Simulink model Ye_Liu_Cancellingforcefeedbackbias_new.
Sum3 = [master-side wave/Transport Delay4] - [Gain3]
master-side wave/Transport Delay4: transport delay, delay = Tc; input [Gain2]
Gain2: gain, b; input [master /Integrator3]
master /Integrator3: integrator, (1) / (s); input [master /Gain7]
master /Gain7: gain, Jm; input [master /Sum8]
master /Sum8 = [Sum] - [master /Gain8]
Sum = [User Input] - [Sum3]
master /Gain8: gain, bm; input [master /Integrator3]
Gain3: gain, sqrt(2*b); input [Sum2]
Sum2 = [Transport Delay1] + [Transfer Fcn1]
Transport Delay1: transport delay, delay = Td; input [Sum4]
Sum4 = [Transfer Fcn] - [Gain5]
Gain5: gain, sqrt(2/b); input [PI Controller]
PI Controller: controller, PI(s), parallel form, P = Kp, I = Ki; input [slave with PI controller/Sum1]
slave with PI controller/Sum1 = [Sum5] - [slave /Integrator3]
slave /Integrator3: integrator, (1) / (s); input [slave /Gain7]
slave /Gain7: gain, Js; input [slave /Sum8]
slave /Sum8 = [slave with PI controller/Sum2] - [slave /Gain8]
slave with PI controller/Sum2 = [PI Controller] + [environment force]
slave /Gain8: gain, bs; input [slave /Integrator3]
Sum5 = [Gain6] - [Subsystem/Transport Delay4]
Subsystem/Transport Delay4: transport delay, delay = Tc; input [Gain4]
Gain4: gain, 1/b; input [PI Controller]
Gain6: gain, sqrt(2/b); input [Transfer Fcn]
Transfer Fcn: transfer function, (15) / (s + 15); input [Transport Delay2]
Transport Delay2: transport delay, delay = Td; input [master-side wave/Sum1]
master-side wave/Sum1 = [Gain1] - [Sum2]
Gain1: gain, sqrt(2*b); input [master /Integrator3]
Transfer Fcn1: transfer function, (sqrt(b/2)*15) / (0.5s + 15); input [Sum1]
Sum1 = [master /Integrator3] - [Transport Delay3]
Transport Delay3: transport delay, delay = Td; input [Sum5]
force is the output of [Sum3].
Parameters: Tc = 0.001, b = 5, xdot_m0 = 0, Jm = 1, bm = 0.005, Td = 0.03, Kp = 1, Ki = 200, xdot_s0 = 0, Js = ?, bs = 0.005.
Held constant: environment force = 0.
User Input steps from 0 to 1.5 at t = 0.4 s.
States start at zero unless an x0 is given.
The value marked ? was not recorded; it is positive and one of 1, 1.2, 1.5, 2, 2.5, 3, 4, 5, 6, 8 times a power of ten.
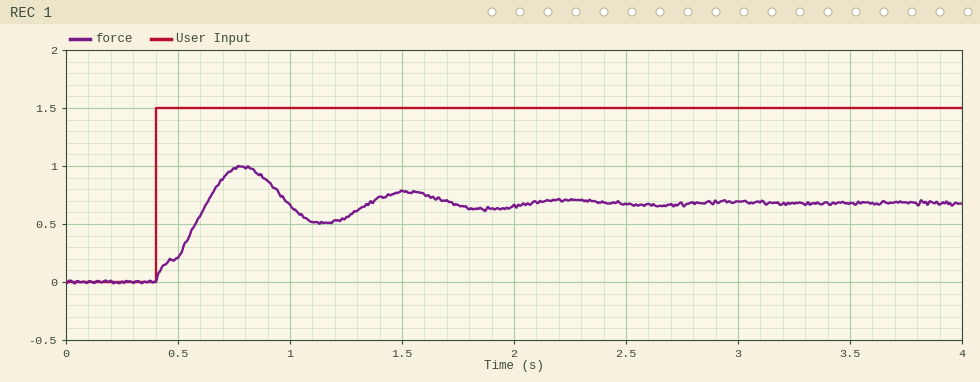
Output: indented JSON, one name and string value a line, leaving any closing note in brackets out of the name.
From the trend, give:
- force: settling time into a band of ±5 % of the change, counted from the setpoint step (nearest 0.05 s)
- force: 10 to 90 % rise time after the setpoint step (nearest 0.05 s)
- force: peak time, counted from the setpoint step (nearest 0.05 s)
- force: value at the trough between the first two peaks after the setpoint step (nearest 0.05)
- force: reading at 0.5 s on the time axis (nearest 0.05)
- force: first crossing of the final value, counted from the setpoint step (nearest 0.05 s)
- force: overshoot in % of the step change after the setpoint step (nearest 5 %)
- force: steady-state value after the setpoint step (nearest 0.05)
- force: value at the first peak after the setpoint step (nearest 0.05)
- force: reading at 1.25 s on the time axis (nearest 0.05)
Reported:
{
  "force: settling time into a band of ±5 % of the change, counted from the setpoint step": "1.60 s",
  "force: 10 to 90 % rise time after the setpoint step": "0.20 s",
  "force: peak time, counted from the setpoint step": "0.40 s",
  "force: value at the trough between the first two peaks after the setpoint step": "0.50",
  "force: reading at 0.5 s on the time axis": "0.20",
  "force: first crossing of the final value, counted from the setpoint step": "0.25 s",
  "force: overshoot in % of the step change after the setpoint step": "45 %",
  "force: steady-state value after the setpoint step": "0.70",
  "force: value at the first peak after the setpoint step": "1.00",
  "force: reading at 1.25 s on the time axis": "0.55"
}
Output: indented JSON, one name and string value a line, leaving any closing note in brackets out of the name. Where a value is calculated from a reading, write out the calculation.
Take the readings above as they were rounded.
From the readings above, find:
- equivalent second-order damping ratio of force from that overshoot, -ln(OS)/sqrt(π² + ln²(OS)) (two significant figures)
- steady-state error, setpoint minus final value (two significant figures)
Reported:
{
  "equivalent second-order damping ratio of force from that overshoot, -ln(OS)/sqrt(π² + ln²(OS))": "ln(0.45) = -0.799; 0.799 / sqrt(9.870 + 0.638) = 0.25",
  "steady-state error, setpoint minus final value": "1.5 - 0.7 = 0.80"
}
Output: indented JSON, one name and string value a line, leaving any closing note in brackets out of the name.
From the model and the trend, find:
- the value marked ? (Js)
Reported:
{
  "the value marked ?": "1.2"
}
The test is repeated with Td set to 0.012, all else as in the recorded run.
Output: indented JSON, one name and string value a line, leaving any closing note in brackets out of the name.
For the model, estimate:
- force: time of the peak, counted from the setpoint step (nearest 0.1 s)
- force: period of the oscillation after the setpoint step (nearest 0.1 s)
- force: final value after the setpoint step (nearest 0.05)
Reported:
{
  "force: time of the peak, counted from the setpoint step": "0.3 s",
  "force: period of the oscillation after the setpoint step": "0.6 s",
  "force: final value after the setpoint step": "0.70"
}
